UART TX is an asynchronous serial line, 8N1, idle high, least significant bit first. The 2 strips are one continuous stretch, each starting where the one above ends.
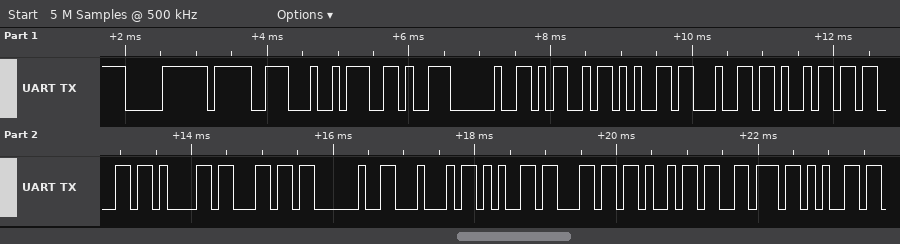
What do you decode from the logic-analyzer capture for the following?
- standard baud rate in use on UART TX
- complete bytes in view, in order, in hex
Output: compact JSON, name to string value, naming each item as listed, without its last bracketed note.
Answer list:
{"standard baud rate in use on UART TX": "9600 baud", "complete bytes in view, in order, in hex": "0xF0 0x9F 0xA4 0x96 0x20 0x4D 0x65 0x64 0x69 0x63 0x61 0x6C 0x20 0x44 0x65 0x6C 0x69 0x76 0x65"}
